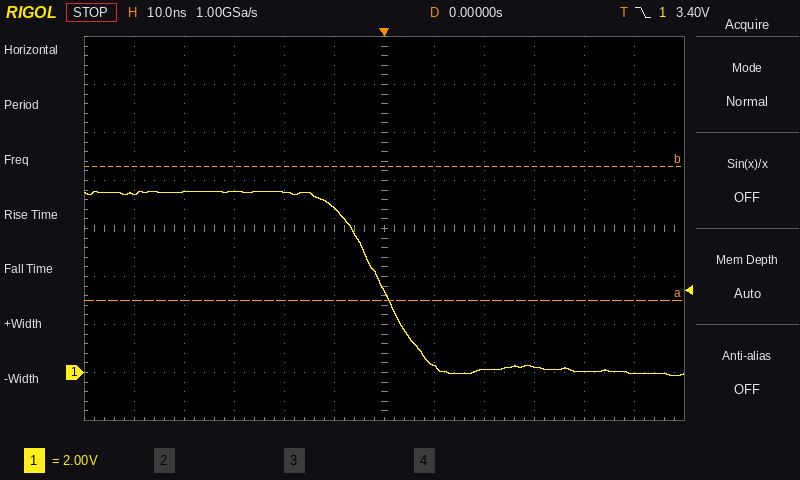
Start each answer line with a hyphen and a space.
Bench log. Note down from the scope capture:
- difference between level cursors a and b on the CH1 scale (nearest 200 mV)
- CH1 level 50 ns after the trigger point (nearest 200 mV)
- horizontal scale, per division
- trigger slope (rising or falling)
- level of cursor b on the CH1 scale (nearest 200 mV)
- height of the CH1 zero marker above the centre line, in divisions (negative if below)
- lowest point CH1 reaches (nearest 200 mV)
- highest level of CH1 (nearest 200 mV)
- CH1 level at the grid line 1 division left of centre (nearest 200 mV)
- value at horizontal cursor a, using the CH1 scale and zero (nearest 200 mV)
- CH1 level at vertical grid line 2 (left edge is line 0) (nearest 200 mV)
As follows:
- 5.6 V
- 0.0 V
- 10 ns
- falling
- 8.6 V
- -3.0 div
- -200 mV
- 7.6 V
- 6.8 V
- 3.0 V
- 7.6 V
